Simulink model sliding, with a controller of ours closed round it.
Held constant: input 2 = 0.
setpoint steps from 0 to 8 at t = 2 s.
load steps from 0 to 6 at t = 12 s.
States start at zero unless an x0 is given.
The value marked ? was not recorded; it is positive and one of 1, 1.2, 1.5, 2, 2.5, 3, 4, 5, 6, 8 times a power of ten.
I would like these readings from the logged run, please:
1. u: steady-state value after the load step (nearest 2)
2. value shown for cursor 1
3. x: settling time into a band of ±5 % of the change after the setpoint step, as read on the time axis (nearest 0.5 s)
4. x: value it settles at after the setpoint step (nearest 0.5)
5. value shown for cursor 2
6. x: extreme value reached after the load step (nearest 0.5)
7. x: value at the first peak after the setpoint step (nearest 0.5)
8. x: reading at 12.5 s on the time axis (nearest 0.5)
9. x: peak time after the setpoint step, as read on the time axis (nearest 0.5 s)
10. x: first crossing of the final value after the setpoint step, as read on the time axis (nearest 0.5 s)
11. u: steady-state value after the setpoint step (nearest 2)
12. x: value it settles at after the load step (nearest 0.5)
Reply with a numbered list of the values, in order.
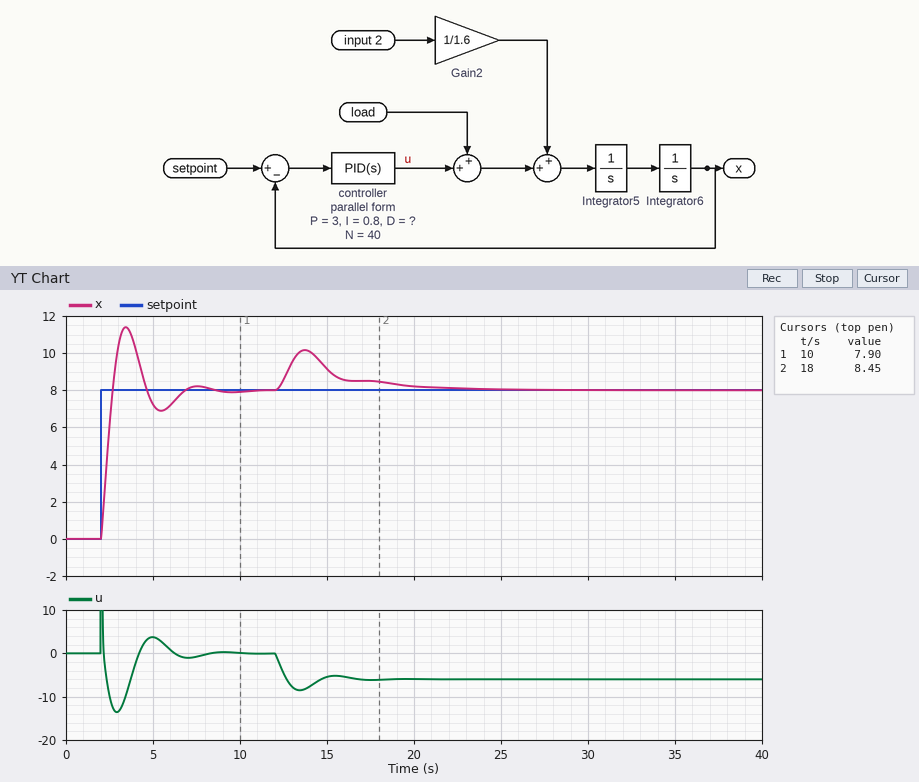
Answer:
1. -6
2. 7.90
3. 6.5 s
4. 8.0
5. 8.45
6. 10.0
7. 11.5
8. 8.5
9. 3.5 s
10. 2.5 s
11. 0
12. 8.0
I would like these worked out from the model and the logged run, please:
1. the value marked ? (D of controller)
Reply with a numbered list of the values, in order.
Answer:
1. 1.5
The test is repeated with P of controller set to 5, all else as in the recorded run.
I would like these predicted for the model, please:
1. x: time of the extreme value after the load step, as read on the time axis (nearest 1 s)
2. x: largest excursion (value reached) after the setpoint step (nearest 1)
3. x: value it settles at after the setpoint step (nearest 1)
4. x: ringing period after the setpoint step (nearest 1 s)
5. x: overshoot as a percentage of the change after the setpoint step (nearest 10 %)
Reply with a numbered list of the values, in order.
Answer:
1. 13 s
2. 12
3. 8
4. 3 s
5. 50 %
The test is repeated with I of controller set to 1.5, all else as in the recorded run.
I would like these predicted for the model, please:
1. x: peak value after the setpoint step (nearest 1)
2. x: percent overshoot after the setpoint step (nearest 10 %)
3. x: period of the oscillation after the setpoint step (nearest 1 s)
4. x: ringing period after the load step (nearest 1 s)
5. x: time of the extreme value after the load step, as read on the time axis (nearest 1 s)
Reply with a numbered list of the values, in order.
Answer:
1. 12
2. 50 %
3. 4 s
4. 4 s
5. 14 s
